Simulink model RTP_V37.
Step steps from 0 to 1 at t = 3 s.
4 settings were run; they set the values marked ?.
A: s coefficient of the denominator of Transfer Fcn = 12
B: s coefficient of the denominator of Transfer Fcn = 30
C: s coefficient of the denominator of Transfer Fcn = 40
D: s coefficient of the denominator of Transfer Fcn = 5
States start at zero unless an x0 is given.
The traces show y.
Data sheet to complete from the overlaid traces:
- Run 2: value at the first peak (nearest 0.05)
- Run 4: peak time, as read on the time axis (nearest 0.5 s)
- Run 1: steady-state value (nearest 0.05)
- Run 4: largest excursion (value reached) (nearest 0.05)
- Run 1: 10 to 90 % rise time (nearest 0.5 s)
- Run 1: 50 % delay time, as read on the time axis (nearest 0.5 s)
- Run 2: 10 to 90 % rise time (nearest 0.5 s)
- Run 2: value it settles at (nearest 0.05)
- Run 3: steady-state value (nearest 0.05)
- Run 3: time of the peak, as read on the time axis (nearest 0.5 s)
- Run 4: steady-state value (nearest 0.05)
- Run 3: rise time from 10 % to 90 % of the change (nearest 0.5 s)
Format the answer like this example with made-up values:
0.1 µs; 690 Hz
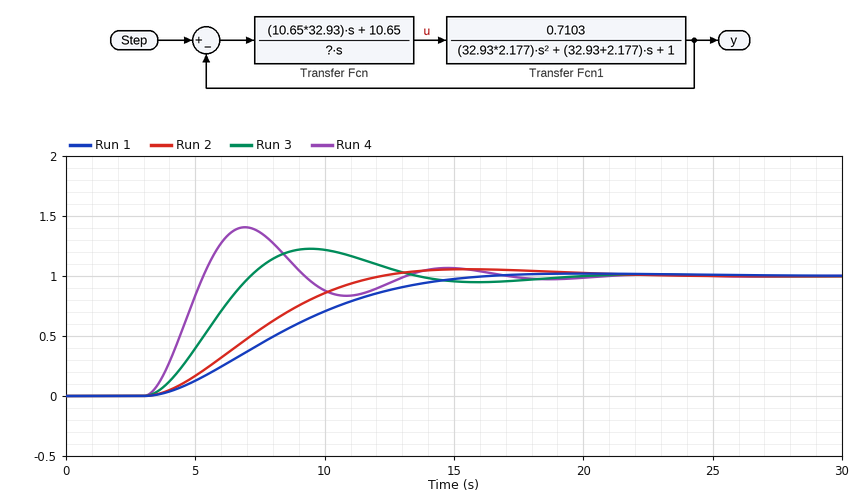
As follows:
1.05; 7.0 s; 1.00; 1.40; 8.0 s; 8.0 s; 6.0 s; 1.00; 1.00; 9.5 s; 1.00; 3.0 s
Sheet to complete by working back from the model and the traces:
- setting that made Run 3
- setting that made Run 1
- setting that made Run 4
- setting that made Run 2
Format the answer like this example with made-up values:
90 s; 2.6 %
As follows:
A; C; D; B
